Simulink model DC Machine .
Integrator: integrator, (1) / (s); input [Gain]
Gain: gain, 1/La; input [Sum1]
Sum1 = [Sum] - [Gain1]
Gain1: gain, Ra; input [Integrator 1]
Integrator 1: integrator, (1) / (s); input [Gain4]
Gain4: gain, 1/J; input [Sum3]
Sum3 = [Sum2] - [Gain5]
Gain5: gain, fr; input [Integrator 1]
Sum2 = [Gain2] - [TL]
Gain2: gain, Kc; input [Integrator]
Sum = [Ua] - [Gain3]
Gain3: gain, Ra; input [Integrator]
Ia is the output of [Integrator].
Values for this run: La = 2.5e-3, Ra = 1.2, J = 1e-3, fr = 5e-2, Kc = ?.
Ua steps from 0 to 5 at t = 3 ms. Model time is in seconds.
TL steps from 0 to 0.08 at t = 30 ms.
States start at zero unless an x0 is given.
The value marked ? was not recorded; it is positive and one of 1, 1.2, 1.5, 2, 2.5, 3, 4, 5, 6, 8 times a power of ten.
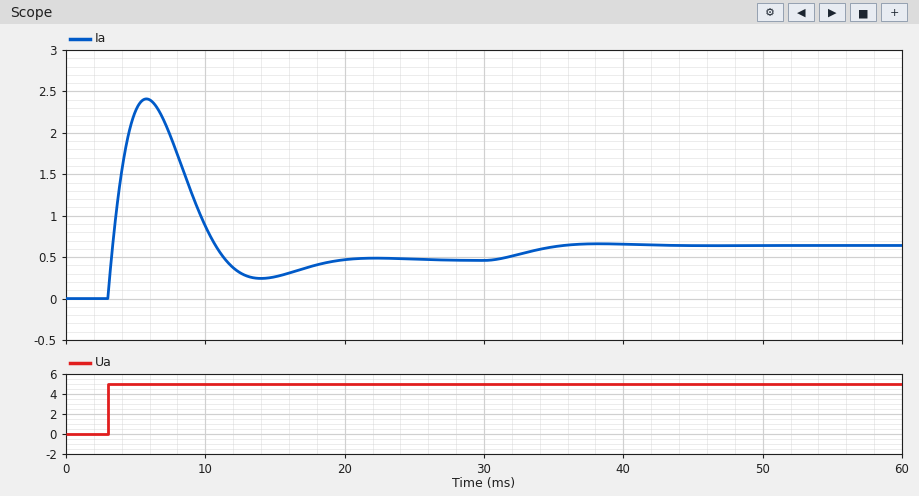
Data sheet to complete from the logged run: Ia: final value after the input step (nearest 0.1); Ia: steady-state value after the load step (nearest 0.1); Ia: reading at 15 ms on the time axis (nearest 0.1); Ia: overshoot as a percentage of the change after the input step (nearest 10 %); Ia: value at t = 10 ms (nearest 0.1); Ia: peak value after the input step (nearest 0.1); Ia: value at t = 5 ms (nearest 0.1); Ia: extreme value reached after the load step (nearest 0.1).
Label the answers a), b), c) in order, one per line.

a) 0.5
b) 0.6
c) 0.3
d) 420 %
e) 0.9
f) 2.4
g) 2.3
h) 0.7
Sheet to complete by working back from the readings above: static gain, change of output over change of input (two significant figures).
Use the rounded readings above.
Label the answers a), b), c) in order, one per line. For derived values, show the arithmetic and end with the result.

a) (0.5 - 0) / (5 - 0) = 0.10
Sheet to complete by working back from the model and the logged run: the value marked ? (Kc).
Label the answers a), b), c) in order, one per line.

a) 0.4
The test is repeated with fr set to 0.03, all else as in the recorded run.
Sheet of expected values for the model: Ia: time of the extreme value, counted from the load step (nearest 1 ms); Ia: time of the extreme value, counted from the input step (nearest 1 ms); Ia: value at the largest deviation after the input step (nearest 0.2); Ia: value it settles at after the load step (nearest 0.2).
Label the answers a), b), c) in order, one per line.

a) 8 ms
b) 3 ms
c) 2.4
d) 0.4
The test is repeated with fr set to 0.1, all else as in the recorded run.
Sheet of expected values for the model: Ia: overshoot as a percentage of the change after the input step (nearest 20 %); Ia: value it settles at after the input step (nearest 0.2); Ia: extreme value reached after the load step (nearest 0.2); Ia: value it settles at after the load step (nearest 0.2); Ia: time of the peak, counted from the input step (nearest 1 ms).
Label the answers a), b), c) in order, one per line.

a) 200 %
b) 0.8
c) 1.0
d) 1.0
e) 3 ms
